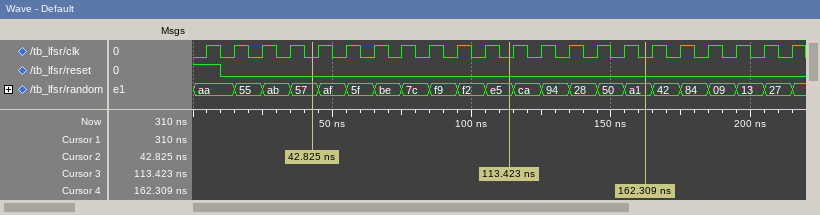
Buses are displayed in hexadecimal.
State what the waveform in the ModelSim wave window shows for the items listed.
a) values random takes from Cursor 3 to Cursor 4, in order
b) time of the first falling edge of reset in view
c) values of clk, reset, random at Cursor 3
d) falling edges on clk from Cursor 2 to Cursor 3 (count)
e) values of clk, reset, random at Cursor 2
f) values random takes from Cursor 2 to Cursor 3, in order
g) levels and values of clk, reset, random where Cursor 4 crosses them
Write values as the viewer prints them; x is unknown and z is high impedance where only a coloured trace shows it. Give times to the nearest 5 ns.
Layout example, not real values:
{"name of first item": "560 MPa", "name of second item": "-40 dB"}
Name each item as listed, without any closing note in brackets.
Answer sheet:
{"values random takes from Cursor 3 to Cursor 4, in order": "e5, ca, 94, 28, 50, a1", "time of the first falling edge of reset in view": "10 ns", "values of clk, reset, random at Cursor 3": "clk=0, reset=0, random=e5", "falling edges on clk from Cursor 2 to Cursor 3": "7", "values of clk, reset, random at Cursor 2": "clk=0, reset=0, random=57", "values random takes from Cursor 2 to Cursor 3, in order": "57, af, 5f, be, 7c, f9, f2, e5", "levels and values of clk, reset, random where Cursor 4 crosses them": "clk=0, reset=0, random=a1"}
